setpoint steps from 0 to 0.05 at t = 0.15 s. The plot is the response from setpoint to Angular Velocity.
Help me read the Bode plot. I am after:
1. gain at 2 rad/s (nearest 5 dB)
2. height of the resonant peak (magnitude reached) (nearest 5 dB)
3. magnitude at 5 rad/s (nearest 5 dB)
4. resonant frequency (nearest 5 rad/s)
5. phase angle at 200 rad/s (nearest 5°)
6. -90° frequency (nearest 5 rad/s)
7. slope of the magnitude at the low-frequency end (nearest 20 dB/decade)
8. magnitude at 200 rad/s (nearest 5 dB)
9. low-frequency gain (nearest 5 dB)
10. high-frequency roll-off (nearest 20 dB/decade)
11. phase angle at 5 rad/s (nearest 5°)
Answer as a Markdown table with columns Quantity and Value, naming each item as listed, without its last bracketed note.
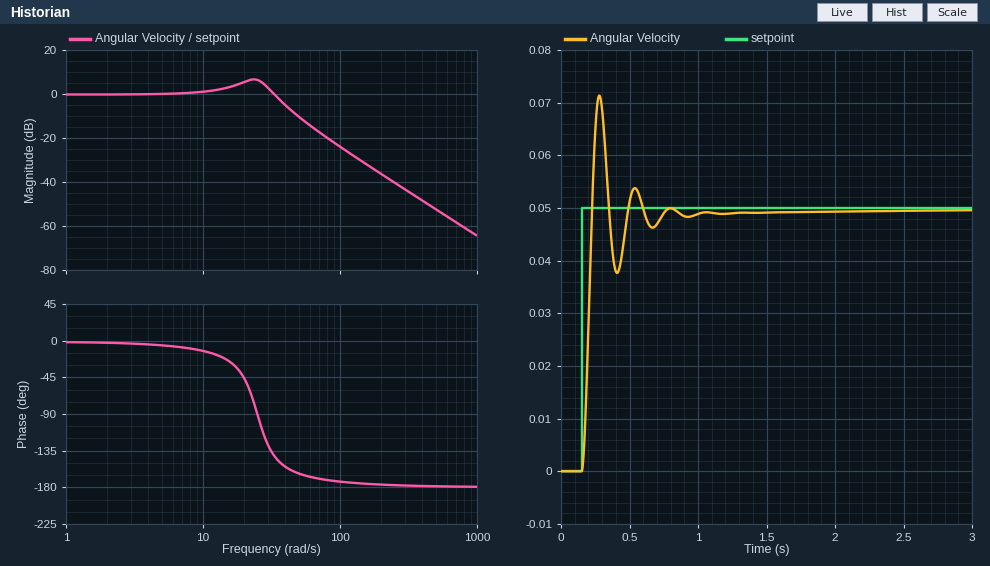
| Quantity | Value |
|---|---|
| gain at 2 rad/s | 0 dB |
| height of the resonant peak (magnitude reached) | 5 dB |
| magnitude at 5 rad/s | 0 dB |
| resonant frequency | 25 rad/s |
| phase angle at 200 rad/s | -175° |
| -90° frequency | 25 rad/s |
| slope of the magnitude at the low-frequency end | 0 dB/decade |
| magnitude at 200 rad/s | -35 dB |
| low-frequency gain | 0 dB |
| high-frequency roll-off | -40 dB/decade |
| phase angle at 5 rad/s | -5° |
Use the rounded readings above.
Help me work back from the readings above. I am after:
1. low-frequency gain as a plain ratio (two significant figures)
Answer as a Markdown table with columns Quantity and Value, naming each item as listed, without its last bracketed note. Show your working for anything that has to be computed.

| Quantity | Value |
|---|---|
| low-frequency gain as a plain ratio | 10^(0 / 20) = 1.0 |
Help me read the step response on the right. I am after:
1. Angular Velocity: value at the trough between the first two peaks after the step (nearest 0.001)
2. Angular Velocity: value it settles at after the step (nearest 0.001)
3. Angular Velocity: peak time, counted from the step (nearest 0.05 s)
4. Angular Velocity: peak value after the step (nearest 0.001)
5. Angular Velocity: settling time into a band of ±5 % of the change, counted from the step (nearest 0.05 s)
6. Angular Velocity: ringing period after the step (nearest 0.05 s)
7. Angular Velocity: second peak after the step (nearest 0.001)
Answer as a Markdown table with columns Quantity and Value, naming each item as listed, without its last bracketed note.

| Quantity | Value |
|---|---|
| Angular Velocity: value at the trough between the first two peaks after the step | 0.038 |
| Angular Velocity: value it settles at after the step | 0.050 |
| Angular Velocity: peak time, counted from the step | 0.15 s |
| Angular Velocity: peak value after the step | 0.071 |
| Angular Velocity: settling time into a band of ±5 % of the change, counted from the step | 0.55 s |
| Angular Velocity: ringing period after the step | 0.25 s |
| Angular Velocity: second peak after the step | 0.054 |
